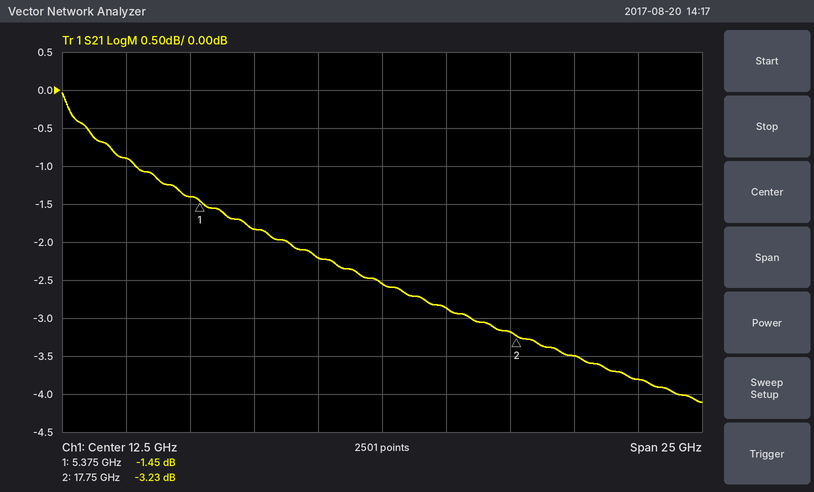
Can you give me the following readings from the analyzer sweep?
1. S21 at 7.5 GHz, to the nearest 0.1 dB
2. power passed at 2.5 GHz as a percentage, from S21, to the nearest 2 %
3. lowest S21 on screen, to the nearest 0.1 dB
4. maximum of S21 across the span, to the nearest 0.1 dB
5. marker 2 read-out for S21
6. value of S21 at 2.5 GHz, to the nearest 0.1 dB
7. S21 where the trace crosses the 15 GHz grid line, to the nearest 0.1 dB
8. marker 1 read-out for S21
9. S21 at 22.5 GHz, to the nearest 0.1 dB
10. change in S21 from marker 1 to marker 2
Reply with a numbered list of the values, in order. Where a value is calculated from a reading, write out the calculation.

1. -1.8 dB
2. 10^(-0.9/10) ≈ 81.3 %, so 82 % to the nearest 2 %
3. -4.1 dB
4. 0.0 dB
5. -3.23 dB
6. -0.9 dB
7. -2.9 dB
8. -1.45 dB
9. -3.8 dB
10. -3.23 − (-1.45) = -1.78 dB
